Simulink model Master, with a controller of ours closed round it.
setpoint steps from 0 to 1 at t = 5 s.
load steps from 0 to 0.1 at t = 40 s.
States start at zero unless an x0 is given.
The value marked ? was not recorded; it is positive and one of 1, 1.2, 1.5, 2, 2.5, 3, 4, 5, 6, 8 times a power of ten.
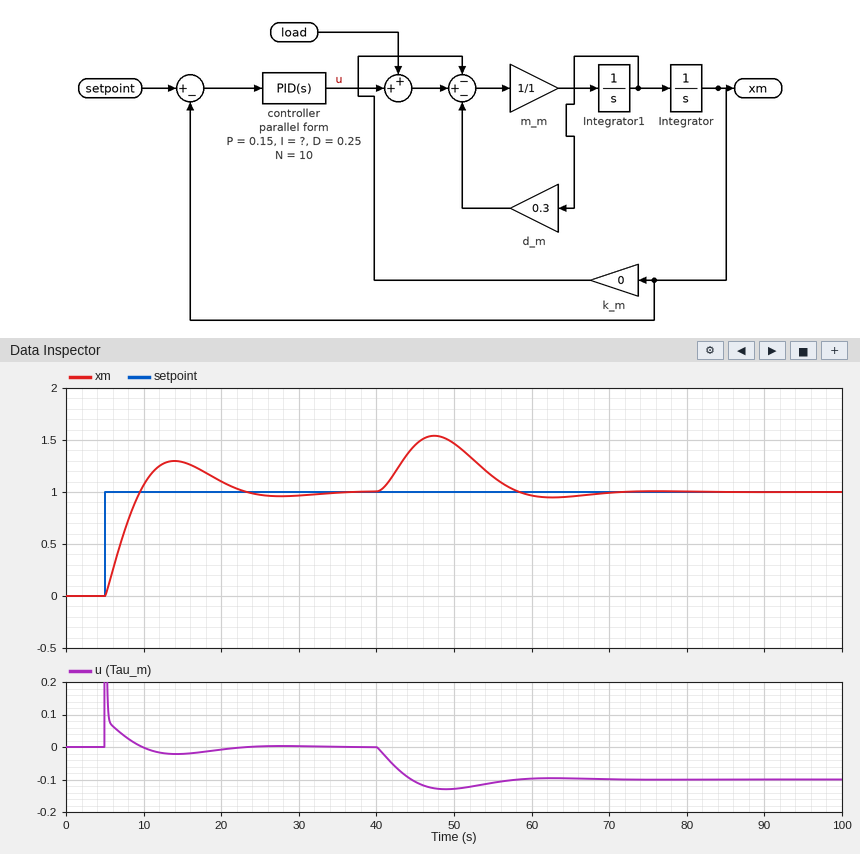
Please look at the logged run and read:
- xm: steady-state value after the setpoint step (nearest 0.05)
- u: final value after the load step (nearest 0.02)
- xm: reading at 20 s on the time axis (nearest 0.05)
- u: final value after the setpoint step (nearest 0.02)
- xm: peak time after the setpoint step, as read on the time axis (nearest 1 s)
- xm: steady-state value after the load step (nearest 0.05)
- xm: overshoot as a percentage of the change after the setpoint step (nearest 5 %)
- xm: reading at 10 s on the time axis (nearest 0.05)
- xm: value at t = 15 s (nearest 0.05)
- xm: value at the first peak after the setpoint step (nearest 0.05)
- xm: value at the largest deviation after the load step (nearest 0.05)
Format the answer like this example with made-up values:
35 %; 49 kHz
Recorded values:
1.00; -0.10; 1.10; 0.00; 14 s; 1.00; 30 %; 1.05; 1.30; 1.30; 1.55
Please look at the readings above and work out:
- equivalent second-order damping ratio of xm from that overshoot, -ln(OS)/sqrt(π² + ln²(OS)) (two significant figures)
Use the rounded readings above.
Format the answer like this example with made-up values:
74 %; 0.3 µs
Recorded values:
0.36
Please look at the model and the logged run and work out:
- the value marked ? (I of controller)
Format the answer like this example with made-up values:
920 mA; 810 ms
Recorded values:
0.02
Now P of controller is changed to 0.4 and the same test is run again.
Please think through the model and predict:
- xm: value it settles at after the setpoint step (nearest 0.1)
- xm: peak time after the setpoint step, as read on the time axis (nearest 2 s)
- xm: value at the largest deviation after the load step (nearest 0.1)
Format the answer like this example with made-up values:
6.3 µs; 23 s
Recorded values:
1.0; 10 s; 1.3
